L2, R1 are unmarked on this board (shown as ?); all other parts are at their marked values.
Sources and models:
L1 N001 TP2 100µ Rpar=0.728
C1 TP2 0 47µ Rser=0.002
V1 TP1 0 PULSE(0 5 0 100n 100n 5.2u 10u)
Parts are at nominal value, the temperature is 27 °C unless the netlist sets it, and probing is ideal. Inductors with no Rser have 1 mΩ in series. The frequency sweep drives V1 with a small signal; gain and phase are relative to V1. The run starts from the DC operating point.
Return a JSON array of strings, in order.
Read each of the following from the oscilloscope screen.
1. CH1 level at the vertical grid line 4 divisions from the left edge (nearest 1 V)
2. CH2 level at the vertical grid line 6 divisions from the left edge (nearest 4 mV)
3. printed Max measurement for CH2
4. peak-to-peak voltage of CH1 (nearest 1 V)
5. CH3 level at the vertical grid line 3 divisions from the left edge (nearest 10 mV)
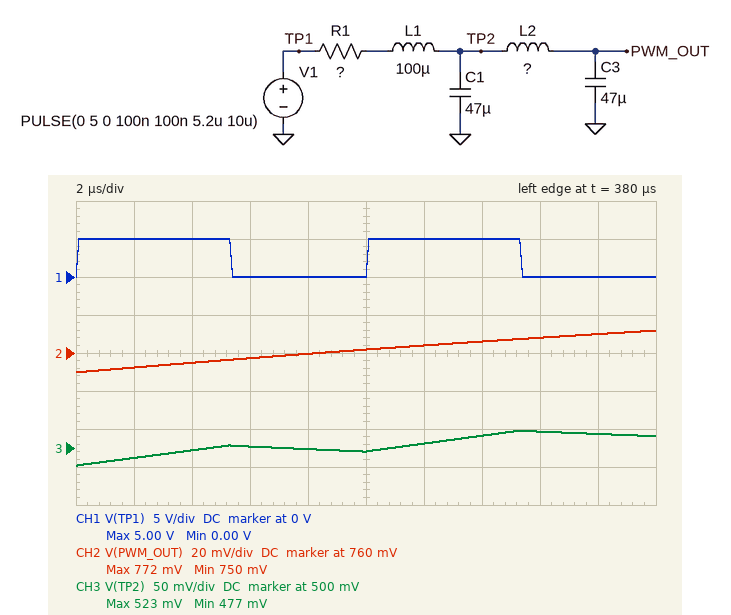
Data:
["0 V", "764 mV", "772 mV", "5 V", "500 mV"]
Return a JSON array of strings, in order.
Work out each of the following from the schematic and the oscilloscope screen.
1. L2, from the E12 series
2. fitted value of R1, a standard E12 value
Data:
["270 µH", "15 Ω"]
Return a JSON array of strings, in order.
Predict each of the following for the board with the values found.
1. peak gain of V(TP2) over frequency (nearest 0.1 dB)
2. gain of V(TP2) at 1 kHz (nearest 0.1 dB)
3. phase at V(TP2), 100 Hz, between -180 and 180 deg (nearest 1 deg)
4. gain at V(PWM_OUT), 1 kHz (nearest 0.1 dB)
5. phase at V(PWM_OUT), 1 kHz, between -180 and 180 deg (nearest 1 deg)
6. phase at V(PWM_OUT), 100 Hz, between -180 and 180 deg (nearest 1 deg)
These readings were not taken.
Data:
["0 dB", "-22.7 dB", "-42 deg", "-16.6 dB", "-87 deg", "-42 deg"]
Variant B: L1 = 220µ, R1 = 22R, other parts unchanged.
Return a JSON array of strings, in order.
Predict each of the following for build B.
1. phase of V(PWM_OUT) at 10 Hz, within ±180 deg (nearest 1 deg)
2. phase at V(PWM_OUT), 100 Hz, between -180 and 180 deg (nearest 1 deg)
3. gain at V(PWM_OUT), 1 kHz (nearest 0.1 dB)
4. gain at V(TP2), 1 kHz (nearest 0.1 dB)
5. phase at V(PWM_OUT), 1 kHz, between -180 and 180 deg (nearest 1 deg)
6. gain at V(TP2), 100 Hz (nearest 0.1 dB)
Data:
["-7 deg", "-53 deg", "-20.0 dB", "-26.0 dB", "-88 deg", "-4.3 dB"]
